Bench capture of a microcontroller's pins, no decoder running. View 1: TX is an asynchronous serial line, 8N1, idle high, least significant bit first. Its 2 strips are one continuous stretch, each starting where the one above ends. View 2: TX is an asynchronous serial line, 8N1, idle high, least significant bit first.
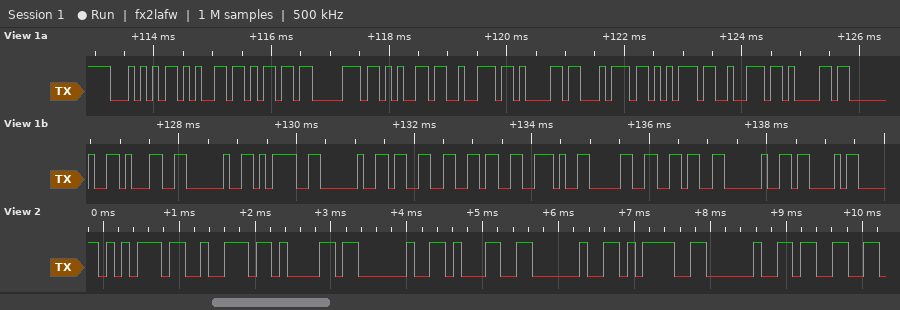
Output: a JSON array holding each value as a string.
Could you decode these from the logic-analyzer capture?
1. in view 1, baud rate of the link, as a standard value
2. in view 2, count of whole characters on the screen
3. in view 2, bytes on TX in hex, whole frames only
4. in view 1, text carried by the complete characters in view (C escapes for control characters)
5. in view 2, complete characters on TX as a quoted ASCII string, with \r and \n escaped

["9600 baud", "9", "75 72 61 20 31 20 3D 20 33", "\"Temperatura 1 = 36.06 C\"", "\"ura 1 = 3\""]
